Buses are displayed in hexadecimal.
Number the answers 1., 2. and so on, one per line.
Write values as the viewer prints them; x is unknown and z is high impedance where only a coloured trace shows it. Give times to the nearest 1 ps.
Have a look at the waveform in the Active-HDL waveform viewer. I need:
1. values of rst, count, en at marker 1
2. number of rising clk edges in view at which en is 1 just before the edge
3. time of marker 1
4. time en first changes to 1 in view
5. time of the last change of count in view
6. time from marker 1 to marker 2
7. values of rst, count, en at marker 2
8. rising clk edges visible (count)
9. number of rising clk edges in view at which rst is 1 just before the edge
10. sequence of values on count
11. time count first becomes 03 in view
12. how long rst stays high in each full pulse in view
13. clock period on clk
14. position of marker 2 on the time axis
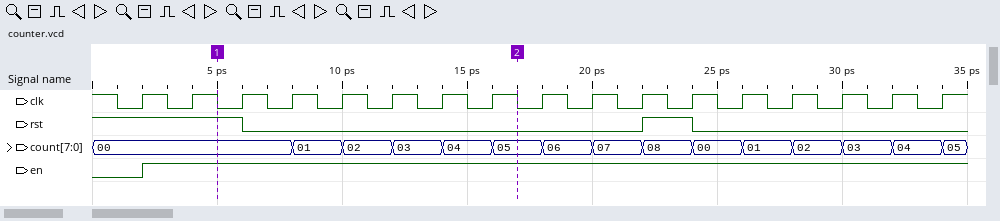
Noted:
1. rst=1, count=00, en=1
2. 16
3. 5 ps
4. 2 ps
5. 34 ps
6. 12 ps
7. rst=0, count=05, en=1
8. 17
9. 4
10. 00, 01, 02, 03, 04, 05, 06, 07, 08, 00, 01, 02, 03, 04, 05
11. 12 ps
12. 2 ps
13. 2 ps
14. 17 ps
